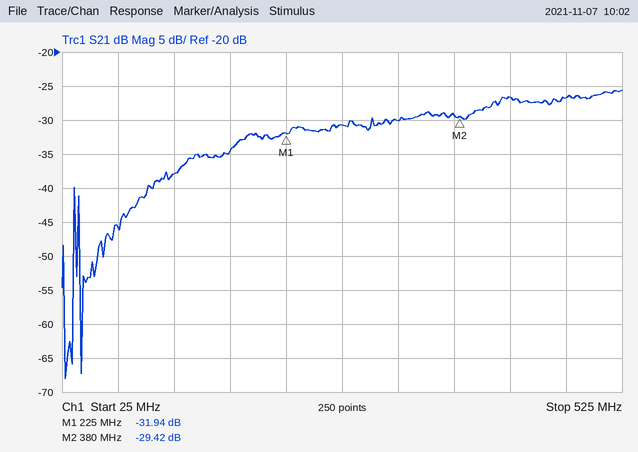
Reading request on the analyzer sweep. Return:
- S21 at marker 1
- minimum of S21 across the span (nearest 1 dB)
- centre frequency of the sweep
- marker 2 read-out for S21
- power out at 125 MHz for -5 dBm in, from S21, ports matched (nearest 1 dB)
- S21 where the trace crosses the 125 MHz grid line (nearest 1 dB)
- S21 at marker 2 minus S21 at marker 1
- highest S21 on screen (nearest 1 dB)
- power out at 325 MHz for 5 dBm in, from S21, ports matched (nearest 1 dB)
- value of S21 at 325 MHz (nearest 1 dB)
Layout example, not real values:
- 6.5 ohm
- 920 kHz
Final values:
- -31.94 dB
- -68 dB
- 275 MHz
- -29.42 dB
- -43 dBm
- -38 dB
- 2.52 dB
- -26 dB
- -25 dBm
- -30 dB
